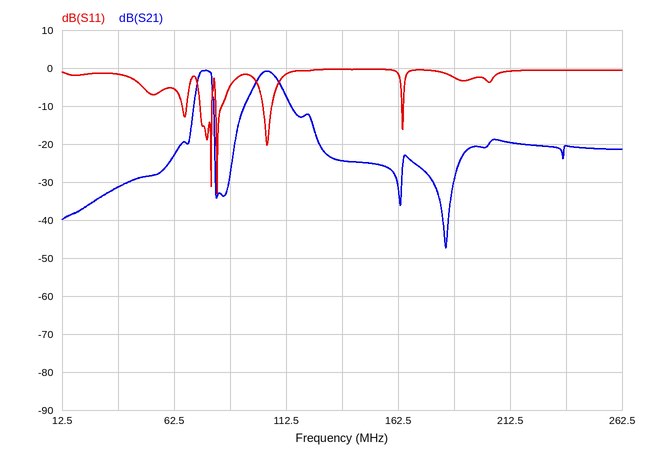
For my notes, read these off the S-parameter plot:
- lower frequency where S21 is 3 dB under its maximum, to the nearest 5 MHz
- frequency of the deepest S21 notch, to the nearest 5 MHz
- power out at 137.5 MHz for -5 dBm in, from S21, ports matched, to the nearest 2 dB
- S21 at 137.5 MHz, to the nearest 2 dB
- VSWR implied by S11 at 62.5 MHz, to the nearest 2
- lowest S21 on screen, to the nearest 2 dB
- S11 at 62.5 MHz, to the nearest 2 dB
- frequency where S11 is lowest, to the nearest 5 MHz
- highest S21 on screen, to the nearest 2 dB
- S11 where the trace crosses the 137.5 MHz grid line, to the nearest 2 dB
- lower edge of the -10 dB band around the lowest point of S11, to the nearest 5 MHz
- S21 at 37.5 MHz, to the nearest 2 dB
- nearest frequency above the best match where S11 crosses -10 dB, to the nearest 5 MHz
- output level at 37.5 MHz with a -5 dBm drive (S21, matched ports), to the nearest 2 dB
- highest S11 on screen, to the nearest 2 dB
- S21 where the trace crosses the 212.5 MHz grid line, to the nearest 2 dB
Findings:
75 MHz
185 MHz
-30 dBm
-24 dB
4
-48 dB
-6 dB
80 MHz
0 dB
0 dB
80 MHz
-32 dB
85 MHz
-36 dBm
0 dB
-20 dB
